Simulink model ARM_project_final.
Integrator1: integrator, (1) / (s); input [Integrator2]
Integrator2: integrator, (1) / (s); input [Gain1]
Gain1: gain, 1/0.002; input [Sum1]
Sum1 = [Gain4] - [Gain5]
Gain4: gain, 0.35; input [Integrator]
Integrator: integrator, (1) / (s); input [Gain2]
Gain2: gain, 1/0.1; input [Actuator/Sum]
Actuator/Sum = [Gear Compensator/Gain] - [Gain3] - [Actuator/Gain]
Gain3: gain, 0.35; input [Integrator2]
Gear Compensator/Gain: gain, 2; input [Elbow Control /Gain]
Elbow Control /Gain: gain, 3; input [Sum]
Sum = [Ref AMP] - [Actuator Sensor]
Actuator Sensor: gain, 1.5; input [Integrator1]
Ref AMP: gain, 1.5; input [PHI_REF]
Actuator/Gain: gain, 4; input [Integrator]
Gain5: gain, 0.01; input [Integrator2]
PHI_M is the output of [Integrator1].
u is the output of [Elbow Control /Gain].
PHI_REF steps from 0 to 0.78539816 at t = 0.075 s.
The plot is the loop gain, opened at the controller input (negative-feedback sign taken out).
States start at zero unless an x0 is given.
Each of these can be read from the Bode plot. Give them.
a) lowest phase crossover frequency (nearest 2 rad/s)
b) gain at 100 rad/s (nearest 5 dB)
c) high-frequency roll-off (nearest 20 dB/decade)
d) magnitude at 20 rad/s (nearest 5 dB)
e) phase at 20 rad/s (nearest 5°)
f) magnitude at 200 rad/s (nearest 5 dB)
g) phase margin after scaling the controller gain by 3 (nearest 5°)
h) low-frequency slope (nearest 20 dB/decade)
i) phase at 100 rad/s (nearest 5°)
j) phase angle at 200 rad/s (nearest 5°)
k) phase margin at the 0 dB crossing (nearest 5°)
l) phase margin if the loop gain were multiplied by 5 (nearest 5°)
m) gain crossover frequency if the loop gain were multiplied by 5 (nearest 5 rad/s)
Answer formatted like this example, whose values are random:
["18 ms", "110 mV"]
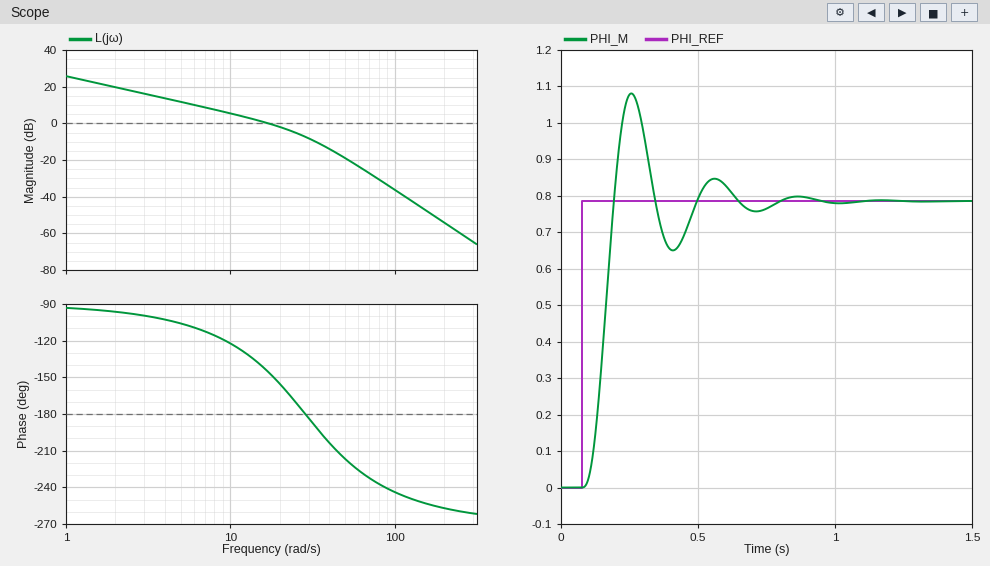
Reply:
["28 rad/s", "-35 dB", "-60 dB/decade", "0 dB", "-155°", "-55 dB", "-10°", "-20 dB/decade", "-245°", "-255°", "35°", "-25°", "40 rad/s"]
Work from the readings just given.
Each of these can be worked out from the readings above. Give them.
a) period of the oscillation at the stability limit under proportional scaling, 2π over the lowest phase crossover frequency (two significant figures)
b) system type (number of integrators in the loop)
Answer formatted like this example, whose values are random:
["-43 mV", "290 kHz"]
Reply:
["0.22 s", "1"]
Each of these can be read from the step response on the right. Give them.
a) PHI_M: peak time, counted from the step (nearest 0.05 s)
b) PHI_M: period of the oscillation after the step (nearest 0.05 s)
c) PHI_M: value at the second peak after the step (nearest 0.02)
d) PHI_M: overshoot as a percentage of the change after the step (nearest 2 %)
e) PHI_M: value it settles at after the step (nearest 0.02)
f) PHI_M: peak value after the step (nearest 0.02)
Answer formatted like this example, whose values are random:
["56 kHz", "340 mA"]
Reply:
["0.20 s", "0.30 s", "0.84", "38 %", "0.78", "1.08"]
